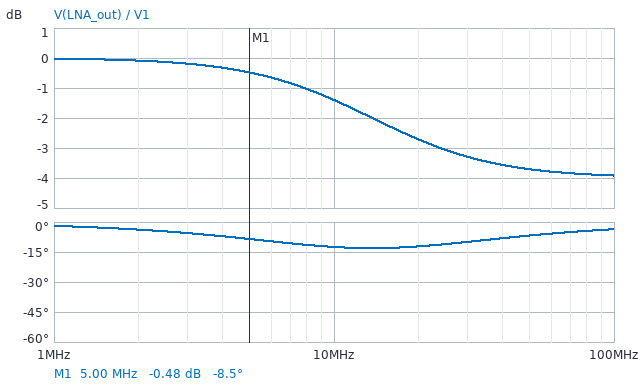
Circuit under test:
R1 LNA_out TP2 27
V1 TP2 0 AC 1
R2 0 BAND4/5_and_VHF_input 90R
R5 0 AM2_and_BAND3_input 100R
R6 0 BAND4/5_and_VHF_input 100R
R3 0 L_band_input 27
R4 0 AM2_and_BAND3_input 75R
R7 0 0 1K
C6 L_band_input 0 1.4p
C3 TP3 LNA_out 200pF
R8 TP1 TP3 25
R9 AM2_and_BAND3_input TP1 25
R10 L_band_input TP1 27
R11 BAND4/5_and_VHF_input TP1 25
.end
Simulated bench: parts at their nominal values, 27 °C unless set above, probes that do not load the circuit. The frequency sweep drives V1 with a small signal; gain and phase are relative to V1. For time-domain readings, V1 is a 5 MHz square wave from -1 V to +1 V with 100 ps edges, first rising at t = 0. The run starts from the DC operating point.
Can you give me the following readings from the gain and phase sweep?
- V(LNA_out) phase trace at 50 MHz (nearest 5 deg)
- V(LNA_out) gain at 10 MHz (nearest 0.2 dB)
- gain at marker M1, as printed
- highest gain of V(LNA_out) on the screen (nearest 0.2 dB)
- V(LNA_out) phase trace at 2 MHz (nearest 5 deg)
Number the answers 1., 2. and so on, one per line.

1. -5 deg
2. -1.4 dB
3. -0.48 dB
4. 0 dB
5. -5 deg
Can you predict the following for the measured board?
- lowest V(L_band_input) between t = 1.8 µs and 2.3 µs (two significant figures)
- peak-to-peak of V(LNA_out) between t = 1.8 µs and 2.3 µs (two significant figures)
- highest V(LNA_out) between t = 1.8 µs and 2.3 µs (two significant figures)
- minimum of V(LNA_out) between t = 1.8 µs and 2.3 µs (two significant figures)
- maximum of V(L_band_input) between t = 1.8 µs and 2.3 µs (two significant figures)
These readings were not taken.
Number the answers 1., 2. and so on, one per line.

1. -290 mV
2. 2.0 V
3. 1.0 V
4. -1.0 V
5. 290 mV
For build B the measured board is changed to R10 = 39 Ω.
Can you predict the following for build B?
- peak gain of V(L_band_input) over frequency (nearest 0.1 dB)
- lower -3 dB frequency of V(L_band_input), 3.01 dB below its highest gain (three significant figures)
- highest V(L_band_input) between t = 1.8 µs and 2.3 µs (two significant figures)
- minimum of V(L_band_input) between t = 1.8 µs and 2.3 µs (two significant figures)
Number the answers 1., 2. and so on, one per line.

1. -18.1 dB
2. 10.6 MHz
3. 250 mV
4. -250 mV
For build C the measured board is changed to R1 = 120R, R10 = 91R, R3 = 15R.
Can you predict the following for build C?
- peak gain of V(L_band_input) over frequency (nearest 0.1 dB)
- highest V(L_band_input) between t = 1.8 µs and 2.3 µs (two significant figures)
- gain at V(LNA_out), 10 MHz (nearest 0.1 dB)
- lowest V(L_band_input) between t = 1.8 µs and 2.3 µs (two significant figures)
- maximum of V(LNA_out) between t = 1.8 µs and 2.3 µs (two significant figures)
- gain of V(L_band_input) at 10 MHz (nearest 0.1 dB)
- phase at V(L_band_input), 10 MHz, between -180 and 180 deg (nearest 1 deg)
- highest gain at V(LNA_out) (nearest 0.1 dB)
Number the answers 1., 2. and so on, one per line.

1. -33.3 dB
2. 41 mV
3. -6.0 dB
4. -41 mV
5. 930 mV
6. -34.1 dB
7. 25 deg
8. 0 dB
